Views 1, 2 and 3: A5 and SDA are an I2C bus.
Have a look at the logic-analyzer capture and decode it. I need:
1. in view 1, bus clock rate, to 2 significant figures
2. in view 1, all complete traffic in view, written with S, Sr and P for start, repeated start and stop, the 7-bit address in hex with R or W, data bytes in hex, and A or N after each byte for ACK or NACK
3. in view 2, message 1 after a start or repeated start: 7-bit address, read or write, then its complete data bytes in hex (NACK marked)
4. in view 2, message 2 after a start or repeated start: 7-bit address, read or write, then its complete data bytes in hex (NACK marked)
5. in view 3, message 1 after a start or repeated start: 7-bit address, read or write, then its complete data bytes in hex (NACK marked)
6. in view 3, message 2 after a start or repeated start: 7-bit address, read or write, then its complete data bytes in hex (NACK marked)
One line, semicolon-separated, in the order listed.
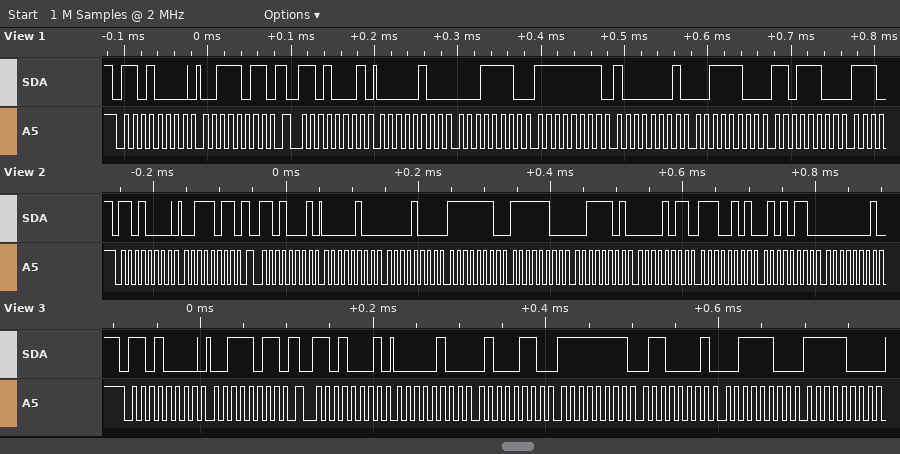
100 kHz; S 68W A 3B A Sr 68R A 04 A 1E A FF A 81 A 3C A DC A; 0x68 write: 3B; 0x68 read: 04 08 FE FC 3D 0B E5 56 01; 0x68 write: 3B; 0x68 read: 04 46 FF 61 3C F8
